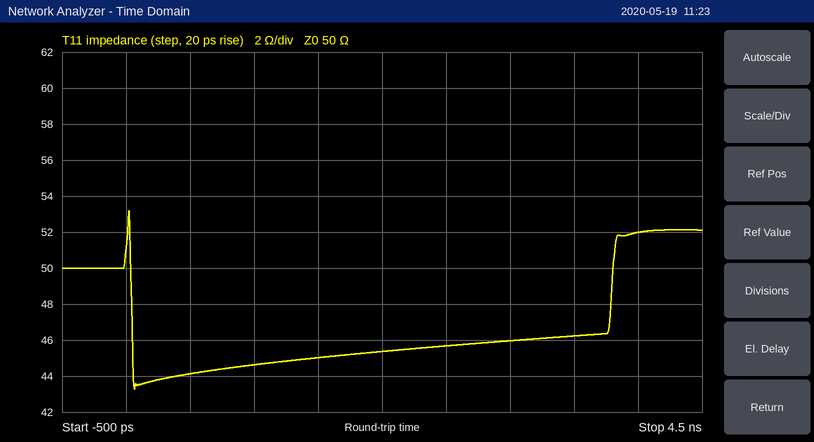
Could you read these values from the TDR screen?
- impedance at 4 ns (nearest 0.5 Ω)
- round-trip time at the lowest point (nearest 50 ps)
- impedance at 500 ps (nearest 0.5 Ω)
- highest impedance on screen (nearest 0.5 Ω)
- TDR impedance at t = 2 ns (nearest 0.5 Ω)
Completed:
52.0 Ω
50 ps
44.0 Ω
53.0 Ω
45.5 Ω
